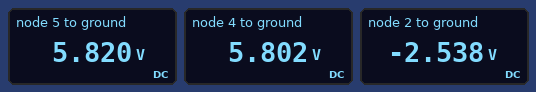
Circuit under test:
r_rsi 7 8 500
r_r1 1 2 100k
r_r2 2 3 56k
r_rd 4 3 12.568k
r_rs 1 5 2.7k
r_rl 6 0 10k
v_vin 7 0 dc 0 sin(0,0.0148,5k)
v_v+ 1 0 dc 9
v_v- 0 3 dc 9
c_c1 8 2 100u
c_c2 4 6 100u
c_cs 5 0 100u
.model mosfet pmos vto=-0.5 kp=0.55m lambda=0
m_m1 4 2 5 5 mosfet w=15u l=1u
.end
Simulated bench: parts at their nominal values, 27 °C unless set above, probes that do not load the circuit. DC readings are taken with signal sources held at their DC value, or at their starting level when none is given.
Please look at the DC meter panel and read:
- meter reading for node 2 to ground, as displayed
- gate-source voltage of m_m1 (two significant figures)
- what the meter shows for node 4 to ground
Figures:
-2.538 V
-8.4 V
5.802 V
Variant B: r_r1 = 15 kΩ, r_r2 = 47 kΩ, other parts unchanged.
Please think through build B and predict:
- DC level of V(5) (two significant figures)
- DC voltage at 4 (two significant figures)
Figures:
5.9 V
5.6 V
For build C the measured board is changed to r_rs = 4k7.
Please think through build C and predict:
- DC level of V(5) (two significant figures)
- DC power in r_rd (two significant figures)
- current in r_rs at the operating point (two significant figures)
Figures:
4.1 V
14 mW
1.0 mA
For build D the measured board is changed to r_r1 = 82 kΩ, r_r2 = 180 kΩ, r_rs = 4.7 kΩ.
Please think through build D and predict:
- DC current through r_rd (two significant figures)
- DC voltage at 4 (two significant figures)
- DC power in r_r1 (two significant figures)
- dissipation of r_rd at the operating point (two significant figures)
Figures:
990 µA
3.4 V
390 µW
12 mW
